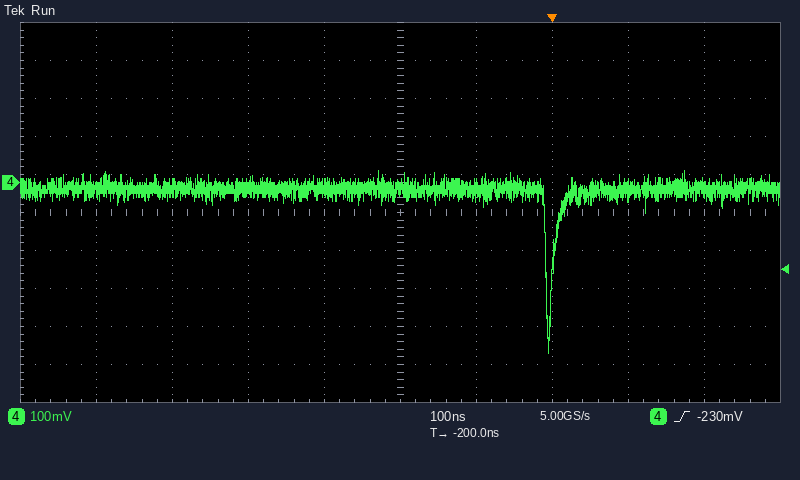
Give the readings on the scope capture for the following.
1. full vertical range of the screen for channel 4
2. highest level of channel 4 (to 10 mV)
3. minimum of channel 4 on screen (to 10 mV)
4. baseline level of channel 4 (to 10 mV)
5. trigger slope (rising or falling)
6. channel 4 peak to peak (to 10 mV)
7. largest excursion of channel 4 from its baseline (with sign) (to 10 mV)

1 V
30 mV
-450 mV
-20 mV
rising
480 mV
-430 mV
